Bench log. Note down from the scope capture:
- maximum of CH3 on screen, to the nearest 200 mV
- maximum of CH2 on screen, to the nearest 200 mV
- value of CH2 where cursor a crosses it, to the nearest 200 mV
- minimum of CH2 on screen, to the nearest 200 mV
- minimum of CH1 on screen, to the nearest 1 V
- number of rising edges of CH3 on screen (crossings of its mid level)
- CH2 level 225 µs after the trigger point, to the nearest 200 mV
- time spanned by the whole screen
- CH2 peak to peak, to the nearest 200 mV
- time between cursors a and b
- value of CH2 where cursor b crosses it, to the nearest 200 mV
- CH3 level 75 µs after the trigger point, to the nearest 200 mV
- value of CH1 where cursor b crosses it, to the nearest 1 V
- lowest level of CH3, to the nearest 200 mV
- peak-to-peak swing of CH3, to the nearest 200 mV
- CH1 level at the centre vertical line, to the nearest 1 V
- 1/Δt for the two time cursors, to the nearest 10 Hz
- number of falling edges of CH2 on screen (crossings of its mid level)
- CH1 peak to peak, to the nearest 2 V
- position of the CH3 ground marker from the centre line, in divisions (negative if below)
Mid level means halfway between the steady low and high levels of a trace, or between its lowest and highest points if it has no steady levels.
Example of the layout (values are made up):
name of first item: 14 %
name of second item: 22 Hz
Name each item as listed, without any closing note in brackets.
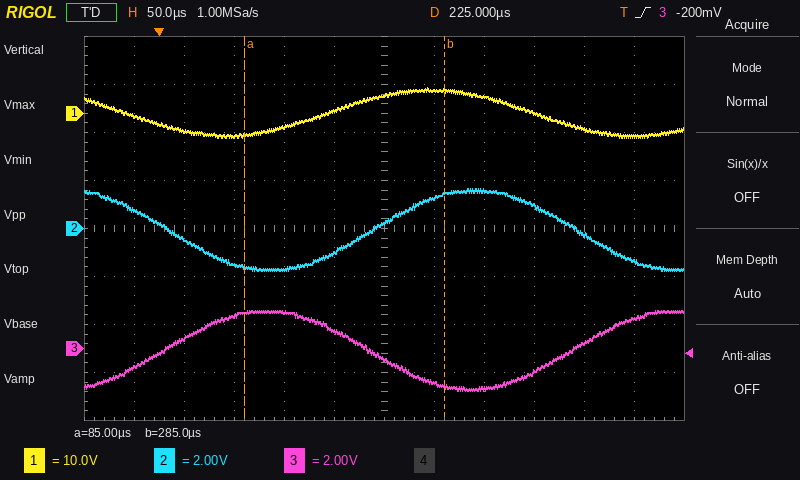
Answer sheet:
maximum of CH3 on screen, to the nearest 200 mV: 1.6 V
maximum of CH2 on screen, to the nearest 200 mV: 1.6 V
value of CH2 where cursor a crosses it, to the nearest 200 mV: -1.6 V
minimum of CH2 on screen, to the nearest 200 mV: -1.8 V
minimum of CH1 on screen, to the nearest 1 V: -5 V
number of rising edges of CH3 on screen: 2
CH2 level 225 µs after the trigger point, to the nearest 200 mV: 200 mV
time spanned by the whole screen: 600 µs
CH2 peak to peak, to the nearest 200 mV: 3.4 V
time between cursors a and b: 200 µs
value of CH2 where cursor b crosses it, to the nearest 200 mV: 1.4 V
CH3 level 75 µs after the trigger point, to the nearest 200 mV: 1.4 V
value of CH1 where cursor b crosses it, to the nearest 1 V: 5 V
lowest level of CH3, to the nearest 200 mV: -1.8 V
peak-to-peak swing of CH3, to the nearest 200 mV: 3.4 V
CH1 level at the centre vertical line, to the nearest 1 V: 4 V
1/Δt for the two time cursors, to the nearest 10 Hz: 5.00 kHz
number of falling edges of CH2 on screen: 2
CH1 peak to peak, to the nearest 2 V: 10 V
position of the CH3 ground marker from the centre line, in divisions: -2.5 div
